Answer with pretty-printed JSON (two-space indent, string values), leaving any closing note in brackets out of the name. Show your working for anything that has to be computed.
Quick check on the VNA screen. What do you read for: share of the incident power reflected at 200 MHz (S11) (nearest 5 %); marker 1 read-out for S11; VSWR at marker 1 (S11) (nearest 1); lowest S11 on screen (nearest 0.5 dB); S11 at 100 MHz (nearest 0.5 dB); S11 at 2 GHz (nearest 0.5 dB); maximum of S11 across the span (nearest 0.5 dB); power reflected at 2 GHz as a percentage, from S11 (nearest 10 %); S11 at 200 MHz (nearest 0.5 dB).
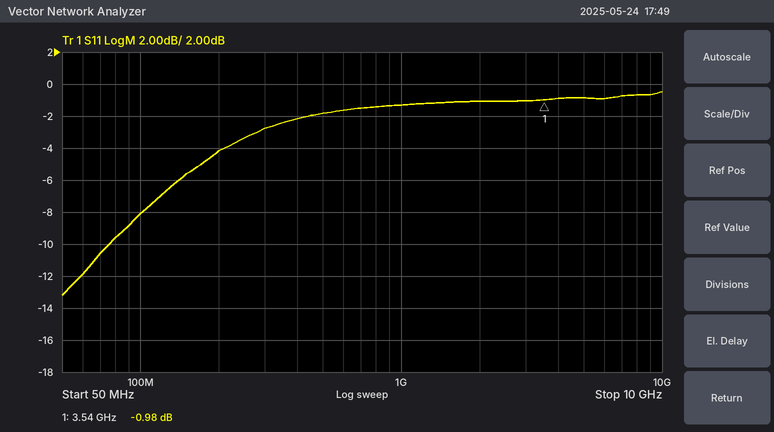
{
  "share of the incident power reflected at 200 MHz (S11)": "10^(-4/10) ≈ 40 %",
  "marker 1 read-out for S11": "-0.98 dB",
  "VSWR at marker 1 (S11)": "(1 + 0.8933)/(1 − 0.8933) ≈ 18",
  "lowest S11 on screen": "-13.0 dB",
  "S11 at 100 MHz": "-8.0 dB",
  "S11 at 2 GHz": "-1.0 dB",
  "maximum of S11 across the span": "-0.5 dB",
  "power reflected at 2 GHz as a percentage, from S11": "10^(-1/10) ≈ 79.4 %, so 80 % to the nearest 10 %",
  "S11 at 200 MHz": "-4.0 dB"
}
